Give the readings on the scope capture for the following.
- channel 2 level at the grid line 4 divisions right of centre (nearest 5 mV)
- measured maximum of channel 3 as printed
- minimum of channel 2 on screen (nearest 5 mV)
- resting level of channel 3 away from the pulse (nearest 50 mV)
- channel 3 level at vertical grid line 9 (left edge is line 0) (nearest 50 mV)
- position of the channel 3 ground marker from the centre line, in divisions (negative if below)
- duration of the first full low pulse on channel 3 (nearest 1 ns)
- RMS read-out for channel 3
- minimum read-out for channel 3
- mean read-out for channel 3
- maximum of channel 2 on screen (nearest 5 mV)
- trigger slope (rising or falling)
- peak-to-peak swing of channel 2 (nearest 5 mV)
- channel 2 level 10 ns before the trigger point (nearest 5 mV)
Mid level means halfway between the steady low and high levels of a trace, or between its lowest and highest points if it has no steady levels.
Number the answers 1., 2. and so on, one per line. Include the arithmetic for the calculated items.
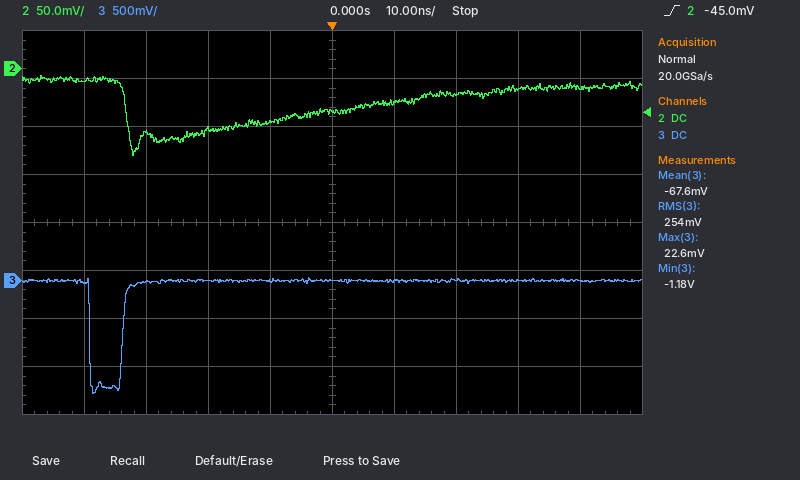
1. -20 mV
2. 22.6 mV
3. -90 mV
4. 0 mV
5. 0 mV
6. -1.2 div
7. 5 ns
8. 254 mV
9. -1.18 V
10. -67.6 mV
11. -5 mV
12. rising
13. -5 mV − (-90 mV) = 85 mV
14. -55 mV
